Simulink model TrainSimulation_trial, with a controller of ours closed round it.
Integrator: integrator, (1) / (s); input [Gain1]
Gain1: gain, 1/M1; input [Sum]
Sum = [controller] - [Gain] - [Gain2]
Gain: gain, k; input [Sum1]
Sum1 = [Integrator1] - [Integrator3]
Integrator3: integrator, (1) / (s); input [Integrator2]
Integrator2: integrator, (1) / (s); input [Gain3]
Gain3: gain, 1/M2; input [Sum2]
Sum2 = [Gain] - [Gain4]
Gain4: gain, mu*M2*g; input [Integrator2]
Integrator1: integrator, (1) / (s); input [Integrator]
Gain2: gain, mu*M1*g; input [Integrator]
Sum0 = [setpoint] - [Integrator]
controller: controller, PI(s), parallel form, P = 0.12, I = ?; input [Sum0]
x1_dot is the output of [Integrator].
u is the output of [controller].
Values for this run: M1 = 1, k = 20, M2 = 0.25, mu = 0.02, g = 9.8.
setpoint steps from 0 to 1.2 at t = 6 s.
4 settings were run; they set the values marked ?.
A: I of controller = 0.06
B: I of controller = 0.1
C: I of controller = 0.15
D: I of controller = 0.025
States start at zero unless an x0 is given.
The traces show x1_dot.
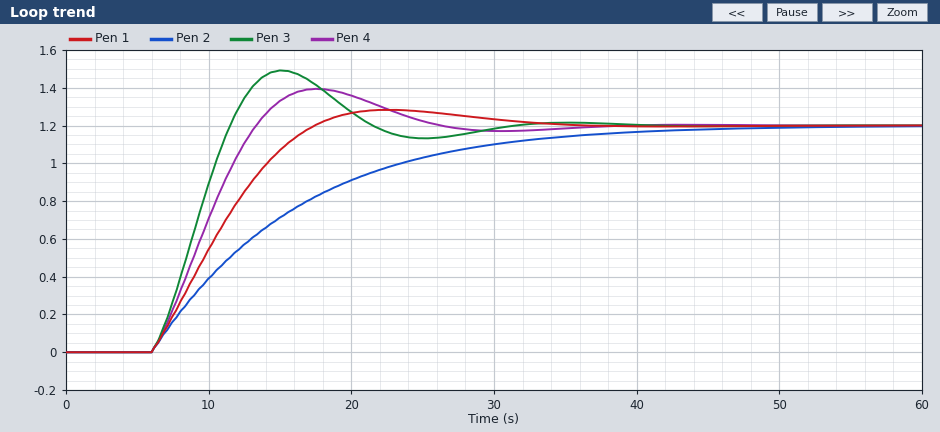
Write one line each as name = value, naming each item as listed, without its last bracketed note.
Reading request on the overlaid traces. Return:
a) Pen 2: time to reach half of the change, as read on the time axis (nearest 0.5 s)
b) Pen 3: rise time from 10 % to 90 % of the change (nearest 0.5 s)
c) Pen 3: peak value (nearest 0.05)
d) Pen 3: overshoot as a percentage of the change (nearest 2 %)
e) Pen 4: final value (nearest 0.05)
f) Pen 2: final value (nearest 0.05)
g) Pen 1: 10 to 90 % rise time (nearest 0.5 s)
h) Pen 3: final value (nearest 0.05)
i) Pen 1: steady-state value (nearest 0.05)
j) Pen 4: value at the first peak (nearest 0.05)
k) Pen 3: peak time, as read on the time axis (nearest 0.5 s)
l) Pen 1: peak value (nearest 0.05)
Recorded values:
Pen 2: time to reach half of the change, as read on the time axis = 13.0 s
Pen 3: rise time from 10 % to 90 % of the change = 4.0 s
Pen 3: peak value = 1.50
Pen 3: overshoot as a percentage of the change = 24 %
Pen 4: final value = 1.20
Pen 2: final value = 1.20
Pen 1: 10 to 90 % rise time = 8.0 s
Pen 3: final value = 1.20
Pen 1: steady-state value = 1.20
Pen 4: value at the first peak = 1.40
Pen 3: peak time, as read on the time axis = 15.0 s
Pen 1: peak value = 1.30
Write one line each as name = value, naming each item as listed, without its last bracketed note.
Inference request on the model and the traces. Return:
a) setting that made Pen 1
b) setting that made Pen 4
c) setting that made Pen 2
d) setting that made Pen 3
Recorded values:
setting that made Pen 1 = A
setting that made Pen 4 = B
setting that made Pen 2 = D
setting that made Pen 3 = C
